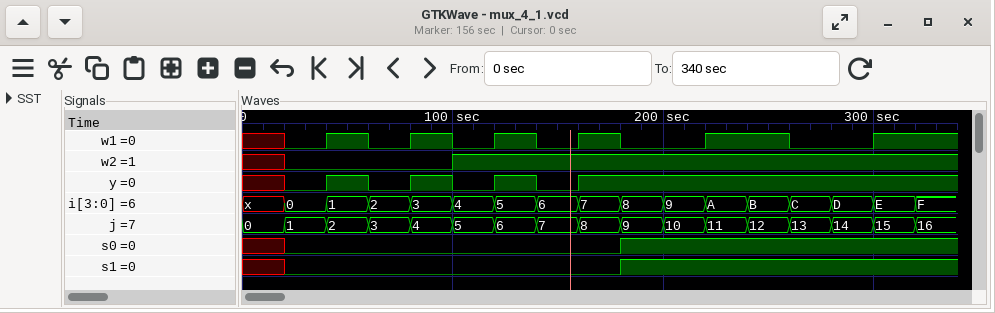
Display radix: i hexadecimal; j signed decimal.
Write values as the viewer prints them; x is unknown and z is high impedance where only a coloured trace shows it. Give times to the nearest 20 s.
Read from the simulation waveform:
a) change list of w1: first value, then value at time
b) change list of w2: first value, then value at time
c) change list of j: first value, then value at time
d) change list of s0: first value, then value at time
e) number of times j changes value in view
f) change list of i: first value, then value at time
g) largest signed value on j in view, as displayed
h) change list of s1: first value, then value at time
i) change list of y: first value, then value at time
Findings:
x, 0 at 20 s, 1 at 40 s, 0 at 60 s, 1 at 80 s, 0 at 100 s, 1 at 120 s, 0 at 140 s, 1 at 160 s, 0 at 180 s, 1 at 220 s, 0 at 260 s, 1 at 300 s
x, 0 at 20 s, 1 at 100 s
0, 1 at 20 s, 2 at 40 s, 3 at 60 s, 4 at 80 s, 5 at 100 s, 6 at 120 s, 7 at 140 s, 8 at 160 s, 9 at 180 s, 10 at 200 s, 11 at 220 s, 12 at 240 s, 13 at 260 s, 14 at 280 s, 15 at 300 s, 16 at 320 s
x, 0 at 20 s, 1 at 180 s
16
x, 0 at 20 s, 1 at 40 s, 2 at 60 s, 3 at 80 s, 4 at 100 s, 5 at 120 s, 6 at 140 s, 7 at 160 s, 8 at 180 s, 9 at 200 s, A at 220 s, B at 240 s, C at 260 s, D at 280 s, E at 300 s, F at 320 s
16
x, 0 at 20 s, 1 at 180 s
x, 0 at 20 s, 1 at 40 s, 0 at 60 s, 1 at 80 s, 0 at 100 s, 1 at 120 s, 0 at 140 s, 1 at 160 s
